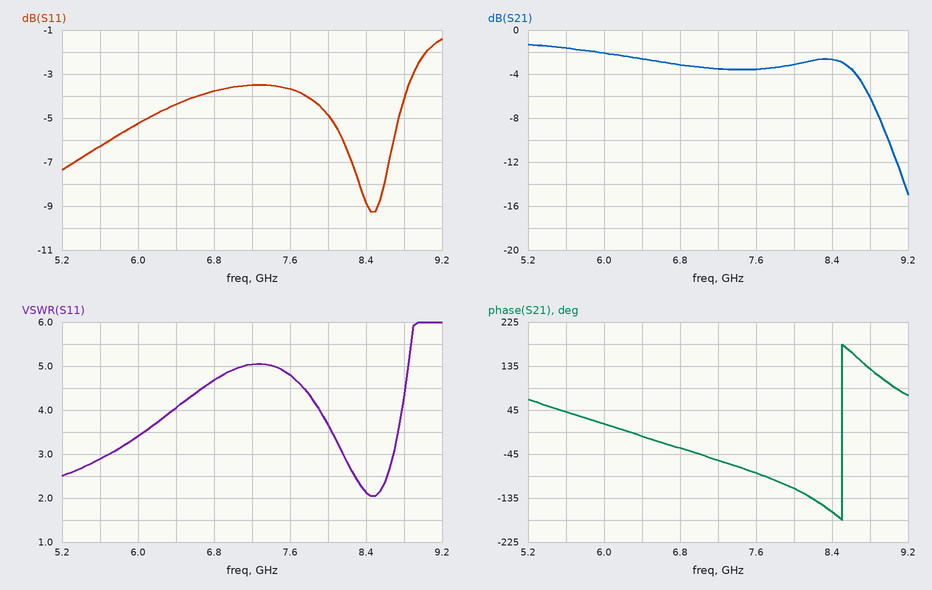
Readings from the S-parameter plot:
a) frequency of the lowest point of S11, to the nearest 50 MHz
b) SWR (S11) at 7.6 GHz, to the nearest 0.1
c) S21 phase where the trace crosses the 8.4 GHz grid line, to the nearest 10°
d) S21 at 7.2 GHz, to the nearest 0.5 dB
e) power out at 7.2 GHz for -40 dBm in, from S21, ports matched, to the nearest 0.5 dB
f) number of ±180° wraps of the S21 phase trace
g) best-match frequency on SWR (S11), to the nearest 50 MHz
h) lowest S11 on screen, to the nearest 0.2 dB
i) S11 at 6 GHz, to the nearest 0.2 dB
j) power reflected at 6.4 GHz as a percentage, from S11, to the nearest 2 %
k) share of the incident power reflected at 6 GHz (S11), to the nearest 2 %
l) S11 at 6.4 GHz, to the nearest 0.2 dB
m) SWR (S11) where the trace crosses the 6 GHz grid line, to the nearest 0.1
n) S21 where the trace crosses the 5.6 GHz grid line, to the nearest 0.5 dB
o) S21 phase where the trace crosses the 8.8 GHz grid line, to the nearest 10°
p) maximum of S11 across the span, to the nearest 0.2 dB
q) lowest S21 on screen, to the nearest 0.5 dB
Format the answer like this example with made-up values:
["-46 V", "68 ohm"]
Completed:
["8.45 GHz", "4.8", "-160°", "-3.5 dB", "-43.5 dBm", "1", "8.45 GHz", "-9.2 dB", "-5.2 dB", "36 %", "30 %", "-4.4 dB", "3.4", "-1.5 dB", "130°", "-1.4 dB", "-15.0 dB"]
